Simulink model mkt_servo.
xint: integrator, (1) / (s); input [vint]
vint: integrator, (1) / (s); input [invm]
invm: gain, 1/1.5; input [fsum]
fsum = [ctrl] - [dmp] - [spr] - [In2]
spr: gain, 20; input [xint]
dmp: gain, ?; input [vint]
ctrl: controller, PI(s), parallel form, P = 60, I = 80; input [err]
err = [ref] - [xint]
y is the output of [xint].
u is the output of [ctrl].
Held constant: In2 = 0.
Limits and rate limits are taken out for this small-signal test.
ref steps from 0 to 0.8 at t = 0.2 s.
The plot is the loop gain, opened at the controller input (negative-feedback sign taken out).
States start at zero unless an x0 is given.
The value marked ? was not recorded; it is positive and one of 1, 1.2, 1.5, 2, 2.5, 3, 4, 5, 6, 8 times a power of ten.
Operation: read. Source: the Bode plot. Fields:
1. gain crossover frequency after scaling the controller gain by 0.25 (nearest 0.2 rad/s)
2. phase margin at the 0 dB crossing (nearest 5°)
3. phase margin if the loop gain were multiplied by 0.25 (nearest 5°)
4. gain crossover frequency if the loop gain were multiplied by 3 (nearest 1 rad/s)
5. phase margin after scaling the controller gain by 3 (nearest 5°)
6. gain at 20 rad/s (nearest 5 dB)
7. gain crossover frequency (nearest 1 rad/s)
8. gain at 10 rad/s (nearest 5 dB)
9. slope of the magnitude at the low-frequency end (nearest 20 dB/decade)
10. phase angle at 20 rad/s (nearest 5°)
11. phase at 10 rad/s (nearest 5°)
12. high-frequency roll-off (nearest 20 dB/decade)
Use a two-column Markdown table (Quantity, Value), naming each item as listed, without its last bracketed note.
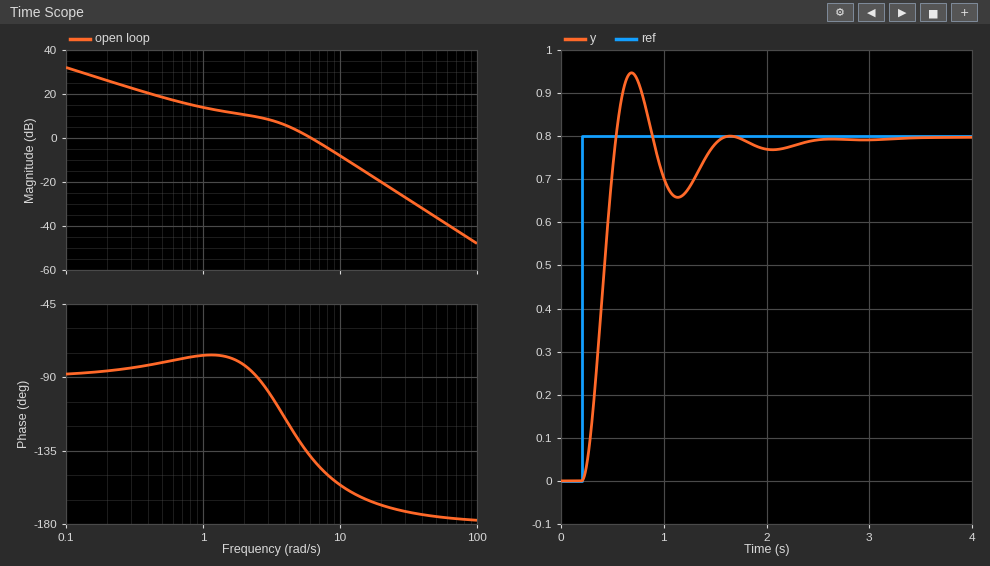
| Quantity | Value |
|---|---|
| gain crossover frequency after scaling the controller gain by 0.25 | 1.4 rad/s |
| phase margin at the 0 dB crossing | 40° |
| phase margin if the loop gain were multiplied by 0.25 | 105° |
| gain crossover frequency if the loop gain were multiplied by 3 | 11 rad/s |
| phase margin after scaling the controller gain by 3 | 20° |
| gain at 20 rad/s | -20 dB |
| gain crossover frequency | 6 rad/s |
| gain at 10 rad/s | -10 dB |
| slope of the magnitude at the low-frequency end | -20 dB/decade |
| phase angle at 20 rad/s | -170° |
| phase at 10 rad/s | -155° |
| high-frequency roll-off | -40 dB/decade |
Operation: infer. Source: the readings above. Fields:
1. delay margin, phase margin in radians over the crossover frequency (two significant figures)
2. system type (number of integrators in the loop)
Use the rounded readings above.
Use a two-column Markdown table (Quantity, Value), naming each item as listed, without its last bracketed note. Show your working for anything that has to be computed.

| Quantity | Value |
|---|---|
| delay margin, phase margin in radians over the crossover frequency | 40 × π / 180 / 6 = 0.12 s |
| system type | 1 |
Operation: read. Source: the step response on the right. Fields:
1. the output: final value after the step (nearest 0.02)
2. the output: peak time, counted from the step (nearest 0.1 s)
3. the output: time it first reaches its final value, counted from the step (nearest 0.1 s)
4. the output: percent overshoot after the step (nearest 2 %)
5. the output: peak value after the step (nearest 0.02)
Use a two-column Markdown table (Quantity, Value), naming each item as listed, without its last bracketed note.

| Quantity | Value |
|---|---|
| the output: final value after the step | 0.80 |
| the output: peak time, counted from the step | 0.5 s |
| the output: time it first reaches its final value, counted from the step | 0.3 s |
| the output: percent overshoot after the step | 18 % |
| the output: peak value after the step | 0.94 |
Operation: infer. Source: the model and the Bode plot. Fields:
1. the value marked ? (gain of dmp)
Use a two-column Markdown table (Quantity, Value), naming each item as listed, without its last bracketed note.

| Quantity | Value |
|---|---|
| the value marked ? | 8 |
